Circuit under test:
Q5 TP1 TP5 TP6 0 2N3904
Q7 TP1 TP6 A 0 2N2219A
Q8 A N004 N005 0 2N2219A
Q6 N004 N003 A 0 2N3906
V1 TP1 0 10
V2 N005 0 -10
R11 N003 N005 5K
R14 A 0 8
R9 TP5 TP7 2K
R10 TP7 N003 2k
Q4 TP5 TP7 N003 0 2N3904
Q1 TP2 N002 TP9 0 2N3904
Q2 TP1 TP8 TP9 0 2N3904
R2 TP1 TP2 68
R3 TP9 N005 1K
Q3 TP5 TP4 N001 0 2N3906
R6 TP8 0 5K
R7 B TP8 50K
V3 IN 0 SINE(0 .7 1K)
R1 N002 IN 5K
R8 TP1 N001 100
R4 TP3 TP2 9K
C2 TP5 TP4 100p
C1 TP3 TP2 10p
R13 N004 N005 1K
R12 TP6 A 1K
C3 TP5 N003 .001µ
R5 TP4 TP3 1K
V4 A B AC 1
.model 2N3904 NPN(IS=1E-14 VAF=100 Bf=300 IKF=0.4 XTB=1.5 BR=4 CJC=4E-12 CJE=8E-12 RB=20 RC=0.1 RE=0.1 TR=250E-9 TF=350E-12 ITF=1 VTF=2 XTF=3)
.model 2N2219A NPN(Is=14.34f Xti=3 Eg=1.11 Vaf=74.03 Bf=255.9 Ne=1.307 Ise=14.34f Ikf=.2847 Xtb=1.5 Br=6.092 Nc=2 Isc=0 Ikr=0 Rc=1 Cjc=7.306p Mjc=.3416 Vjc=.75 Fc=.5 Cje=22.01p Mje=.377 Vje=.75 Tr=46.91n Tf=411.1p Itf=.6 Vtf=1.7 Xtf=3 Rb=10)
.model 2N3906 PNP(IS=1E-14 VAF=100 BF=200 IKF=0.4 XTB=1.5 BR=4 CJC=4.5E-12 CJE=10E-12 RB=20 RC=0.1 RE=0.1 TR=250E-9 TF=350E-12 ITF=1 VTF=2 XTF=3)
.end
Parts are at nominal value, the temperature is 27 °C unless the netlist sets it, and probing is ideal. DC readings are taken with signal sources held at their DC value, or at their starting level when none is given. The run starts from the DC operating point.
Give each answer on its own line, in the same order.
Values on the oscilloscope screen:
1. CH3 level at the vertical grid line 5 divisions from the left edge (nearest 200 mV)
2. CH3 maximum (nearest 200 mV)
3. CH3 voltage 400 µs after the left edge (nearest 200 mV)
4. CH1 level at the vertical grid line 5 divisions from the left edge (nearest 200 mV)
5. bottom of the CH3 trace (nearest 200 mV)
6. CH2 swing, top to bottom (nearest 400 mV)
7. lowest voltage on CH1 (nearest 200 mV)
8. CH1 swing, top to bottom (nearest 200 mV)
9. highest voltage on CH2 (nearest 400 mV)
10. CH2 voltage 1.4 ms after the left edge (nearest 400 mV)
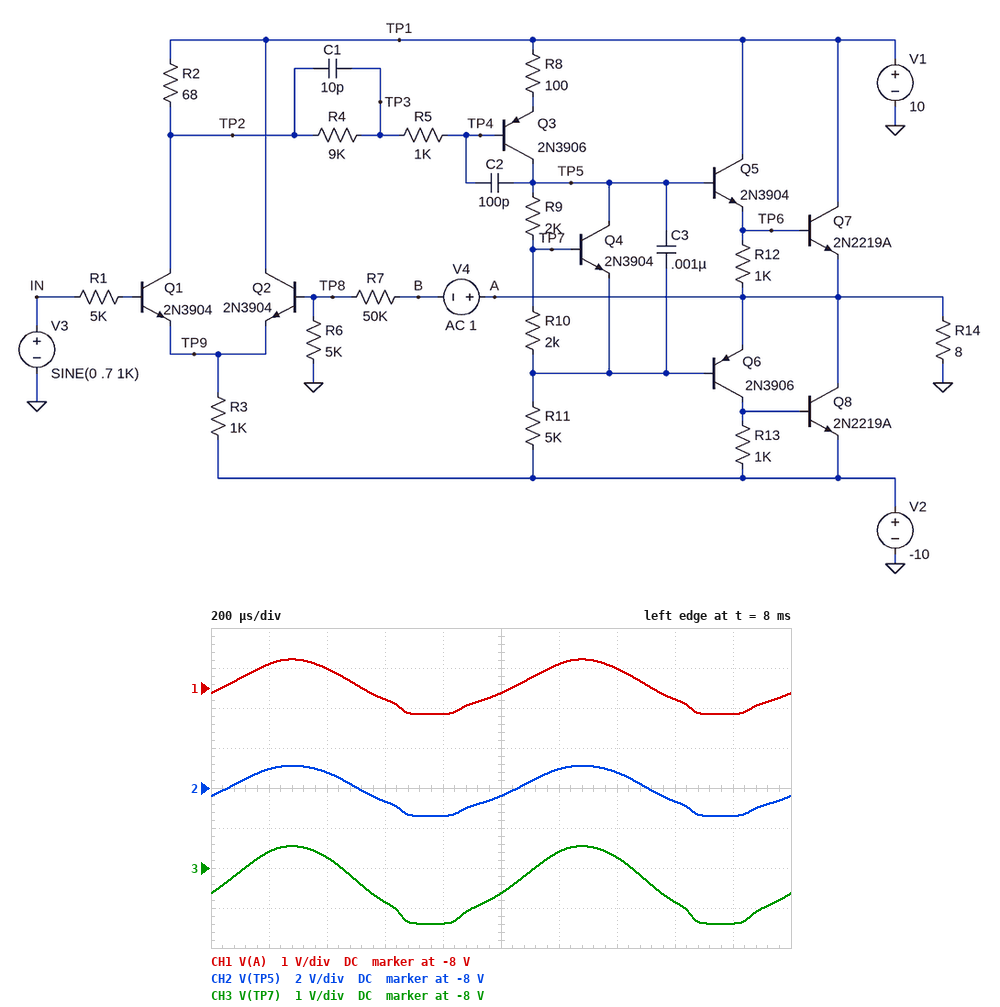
-8.6 V
-7.4 V
-7.8 V
-8.2 V
-9.4 V
2.4 V
-8.6 V
1.4 V
-6.8 V
-7.2 V
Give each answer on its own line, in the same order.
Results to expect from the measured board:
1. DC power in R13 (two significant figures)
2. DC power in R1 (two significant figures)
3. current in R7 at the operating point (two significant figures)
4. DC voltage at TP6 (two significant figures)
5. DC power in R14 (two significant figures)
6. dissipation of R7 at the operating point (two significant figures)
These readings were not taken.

1.1 mW
4.0 µW
150 µA
-8.0 V
8.1 W
1.1 mW
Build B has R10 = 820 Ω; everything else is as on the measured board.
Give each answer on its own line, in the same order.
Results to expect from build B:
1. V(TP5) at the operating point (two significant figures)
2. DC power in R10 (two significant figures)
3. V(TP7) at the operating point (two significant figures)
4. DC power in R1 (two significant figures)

-8.4 V
16 µW
-8.7 V
4.0 µW
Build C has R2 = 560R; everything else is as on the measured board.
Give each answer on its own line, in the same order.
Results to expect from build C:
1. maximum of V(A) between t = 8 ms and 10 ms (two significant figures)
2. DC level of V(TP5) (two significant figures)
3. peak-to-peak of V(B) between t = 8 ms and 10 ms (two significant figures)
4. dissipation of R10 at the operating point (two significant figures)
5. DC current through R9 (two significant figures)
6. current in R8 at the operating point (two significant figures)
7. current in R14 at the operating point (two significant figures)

7.8 V
2.7 V
14 V
230 µW
340 µA
2.3 mA
160 mA
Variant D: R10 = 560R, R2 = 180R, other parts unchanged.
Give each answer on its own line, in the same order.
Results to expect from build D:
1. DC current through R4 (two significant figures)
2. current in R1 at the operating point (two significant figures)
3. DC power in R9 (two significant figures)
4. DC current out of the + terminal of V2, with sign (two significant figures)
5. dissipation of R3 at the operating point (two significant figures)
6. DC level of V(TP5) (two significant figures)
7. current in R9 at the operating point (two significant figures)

7.9 µA
16 µA
2.5 mW
-1.9 A
85 mW
1.8 V
1.1 mA
